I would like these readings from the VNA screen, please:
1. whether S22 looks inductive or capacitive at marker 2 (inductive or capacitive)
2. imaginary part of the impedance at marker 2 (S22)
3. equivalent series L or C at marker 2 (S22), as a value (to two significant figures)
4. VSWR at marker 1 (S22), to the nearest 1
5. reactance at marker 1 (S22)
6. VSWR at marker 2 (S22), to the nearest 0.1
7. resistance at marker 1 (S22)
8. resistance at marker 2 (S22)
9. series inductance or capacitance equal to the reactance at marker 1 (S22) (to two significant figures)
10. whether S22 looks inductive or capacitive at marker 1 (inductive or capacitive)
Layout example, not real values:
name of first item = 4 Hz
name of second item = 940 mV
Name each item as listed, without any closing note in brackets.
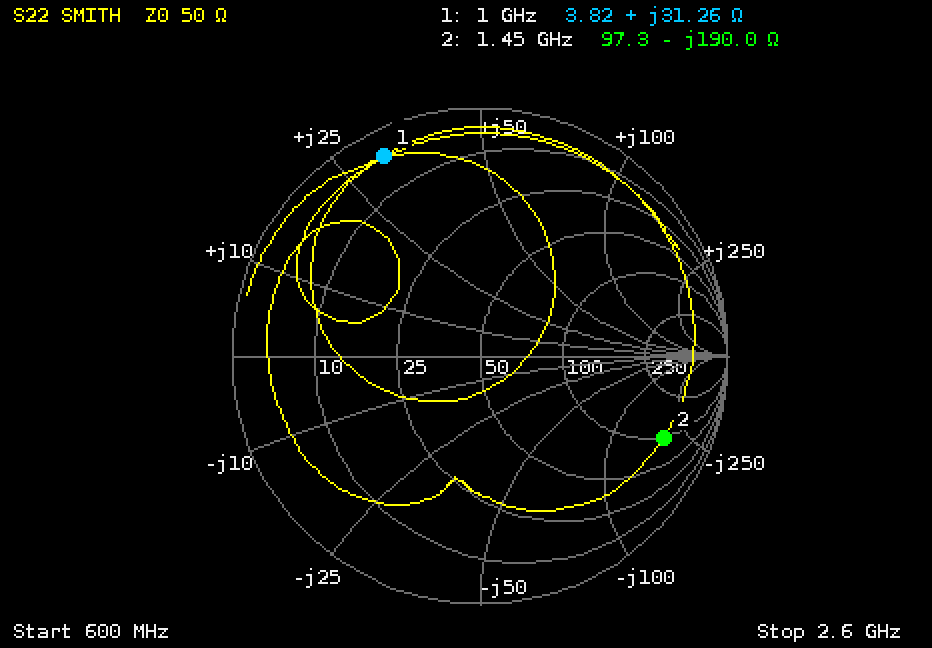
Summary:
whether S22 looks inductive or capacitive at marker 2 = capacitive
imaginary part of the impedance at marker 2 = -190.0 Ω
equivalent series L or C at marker 2 (S22), as a value = 580 fF
VSWR at marker 1 (S22), to the nearest 1 = 18
reactance at marker 1 = +31.26 Ω
VSWR at marker 2 (S22), to the nearest 0.1 = 9.8
resistance at marker 1 = 3.82 Ω
resistance at marker 2 = 97.3 Ω
series inductance or capacitance equal to the reactance at marker 1 (S22) = 5.0 nH
whether S22 looks inductive or capacitive at marker 1 = inductive
